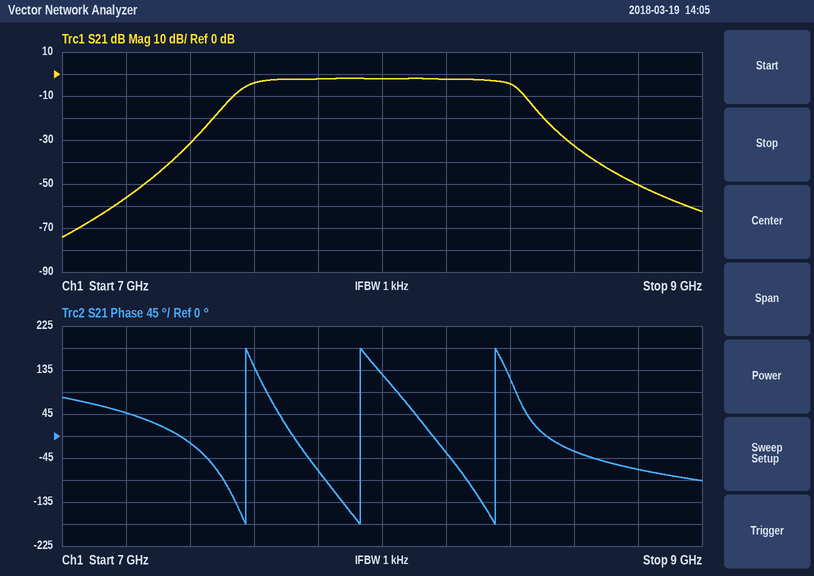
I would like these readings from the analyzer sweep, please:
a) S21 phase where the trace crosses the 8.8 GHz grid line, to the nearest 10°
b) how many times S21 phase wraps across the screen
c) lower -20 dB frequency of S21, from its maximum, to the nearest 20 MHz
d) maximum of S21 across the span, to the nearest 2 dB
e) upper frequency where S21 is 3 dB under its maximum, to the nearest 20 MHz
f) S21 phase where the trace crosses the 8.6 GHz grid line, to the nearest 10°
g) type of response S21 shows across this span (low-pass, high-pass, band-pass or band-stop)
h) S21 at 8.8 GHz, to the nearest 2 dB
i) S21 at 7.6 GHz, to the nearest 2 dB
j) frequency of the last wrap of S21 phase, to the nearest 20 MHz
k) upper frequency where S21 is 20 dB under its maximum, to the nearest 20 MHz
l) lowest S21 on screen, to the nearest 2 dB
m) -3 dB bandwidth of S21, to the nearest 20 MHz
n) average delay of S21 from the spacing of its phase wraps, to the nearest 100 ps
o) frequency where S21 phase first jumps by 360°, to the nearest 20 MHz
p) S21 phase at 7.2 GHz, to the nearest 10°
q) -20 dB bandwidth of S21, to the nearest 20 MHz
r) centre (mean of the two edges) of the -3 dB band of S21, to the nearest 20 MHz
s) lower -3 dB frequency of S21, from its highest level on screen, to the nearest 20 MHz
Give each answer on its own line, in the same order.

-70°
3
7.46 GHz
-2 dB
8.40 GHz
-30°
band-pass
-50 dB
-4 dB
8.36 GHz
8.52 GHz
-74 dB
820 MHz
2.6 ns
7.58 GHz
50°
1.06 GHz
8.00 GHz
7.58 GHz
